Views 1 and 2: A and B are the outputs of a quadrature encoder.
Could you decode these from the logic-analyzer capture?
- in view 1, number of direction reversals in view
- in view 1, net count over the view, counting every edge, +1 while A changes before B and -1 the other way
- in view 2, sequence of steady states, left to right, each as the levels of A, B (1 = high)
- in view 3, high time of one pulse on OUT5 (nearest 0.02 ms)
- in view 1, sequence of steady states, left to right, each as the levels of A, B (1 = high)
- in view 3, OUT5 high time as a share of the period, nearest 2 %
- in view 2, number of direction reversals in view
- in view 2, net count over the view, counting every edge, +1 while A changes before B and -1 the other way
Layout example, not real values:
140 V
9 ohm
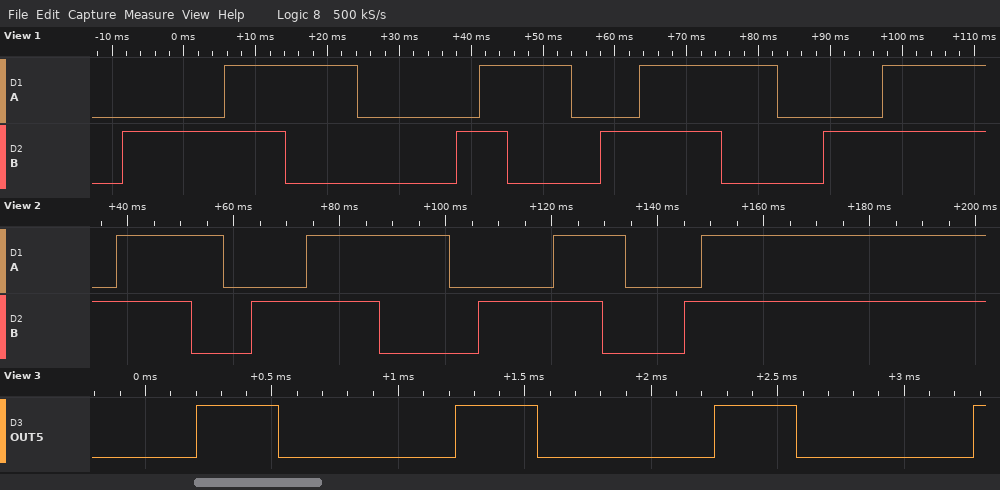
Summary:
0
-14
01 11 10 00 01 11 10 00 01 11 10 00 01 11
0.32 ms
00 01 11 10 00 01 11 10 00 01 11 10 00 01 11
32 %
0
-13
